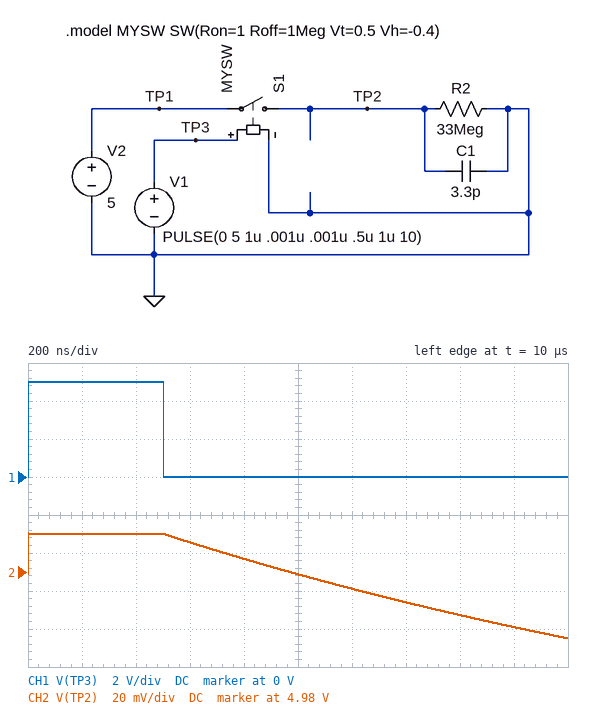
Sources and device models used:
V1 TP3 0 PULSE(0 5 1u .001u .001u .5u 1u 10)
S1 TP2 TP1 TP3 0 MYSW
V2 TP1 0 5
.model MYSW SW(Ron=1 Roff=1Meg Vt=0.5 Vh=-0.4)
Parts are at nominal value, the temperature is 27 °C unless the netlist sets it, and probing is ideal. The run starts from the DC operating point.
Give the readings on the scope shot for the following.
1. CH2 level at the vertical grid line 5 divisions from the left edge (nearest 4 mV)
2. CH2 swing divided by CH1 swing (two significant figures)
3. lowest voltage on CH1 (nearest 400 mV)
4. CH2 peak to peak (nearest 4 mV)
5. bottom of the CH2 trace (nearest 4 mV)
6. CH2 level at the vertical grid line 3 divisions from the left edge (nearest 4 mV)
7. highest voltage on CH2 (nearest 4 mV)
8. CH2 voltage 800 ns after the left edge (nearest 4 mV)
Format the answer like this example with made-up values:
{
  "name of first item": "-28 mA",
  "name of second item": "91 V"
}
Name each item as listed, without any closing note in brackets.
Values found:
{
  "CH2 level at the vertical grid line 5 divisions from the left edge": "4.980 V",
  "CH2 swing divided by CH1 swing": "0.011",
  "lowest voltage on CH1": "0 V",
  "CH2 peak to peak": "56 mV",
  "bottom of the CH2 trace": "4.944 V",
  "CH2 level at the vertical grid line 3 divisions from the left edge": "4.996 V",
  "highest voltage on CH2": "5.000 V",
  "CH2 voltage 800 ns after the left edge": "4.988 V"
}
